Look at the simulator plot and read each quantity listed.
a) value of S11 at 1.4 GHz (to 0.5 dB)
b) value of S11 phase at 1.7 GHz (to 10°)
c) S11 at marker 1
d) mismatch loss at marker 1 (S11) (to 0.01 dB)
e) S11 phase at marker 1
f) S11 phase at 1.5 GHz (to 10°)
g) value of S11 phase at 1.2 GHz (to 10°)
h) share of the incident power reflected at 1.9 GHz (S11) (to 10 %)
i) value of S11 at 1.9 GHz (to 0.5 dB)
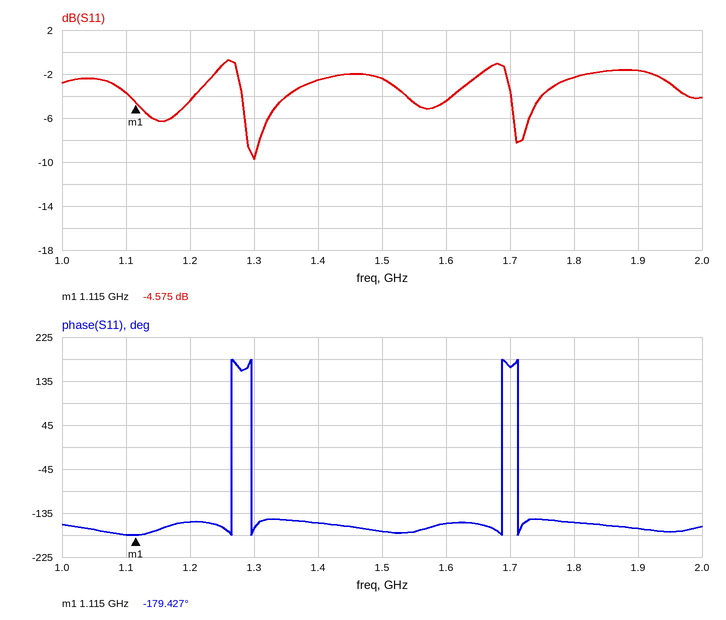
-2.5 dB
160°
-4.575 dB
1.86 dB
-179.427°
-170°
-150°
70 %
-1.5 dB
